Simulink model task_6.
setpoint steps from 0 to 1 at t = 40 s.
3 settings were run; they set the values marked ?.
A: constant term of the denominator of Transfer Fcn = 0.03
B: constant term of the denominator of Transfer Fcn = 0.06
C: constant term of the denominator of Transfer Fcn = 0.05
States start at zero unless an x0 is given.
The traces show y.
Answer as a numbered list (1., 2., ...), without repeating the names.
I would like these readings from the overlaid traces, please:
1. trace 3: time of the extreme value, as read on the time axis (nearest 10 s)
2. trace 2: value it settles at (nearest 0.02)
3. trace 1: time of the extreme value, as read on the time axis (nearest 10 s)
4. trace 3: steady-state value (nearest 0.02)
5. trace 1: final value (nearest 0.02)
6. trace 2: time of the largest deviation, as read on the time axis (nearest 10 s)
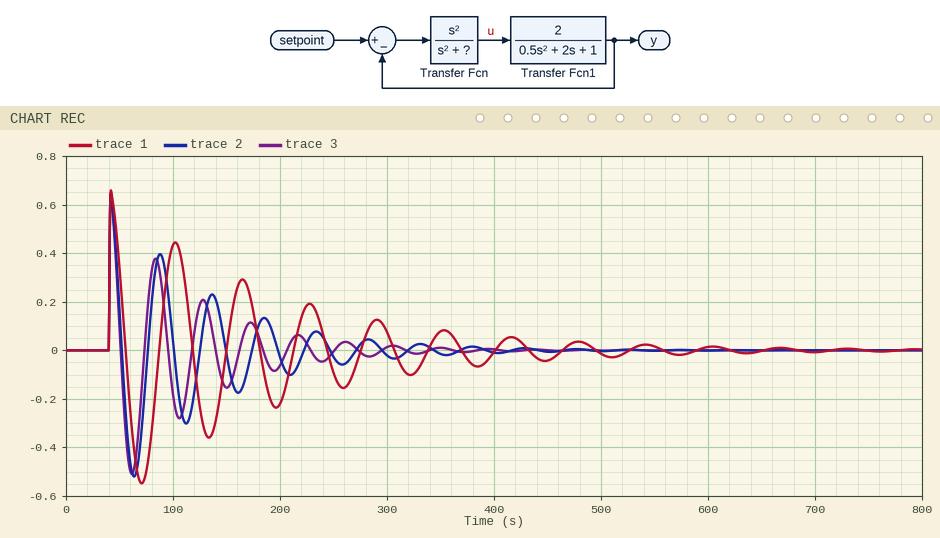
1. 40 s
2. 0.00
3. 40 s
4. 0.00
5. 0.00
6. 40 s
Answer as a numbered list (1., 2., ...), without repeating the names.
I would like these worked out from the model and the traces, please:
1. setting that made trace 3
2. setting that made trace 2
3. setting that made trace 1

1. B
2. C
3. A
